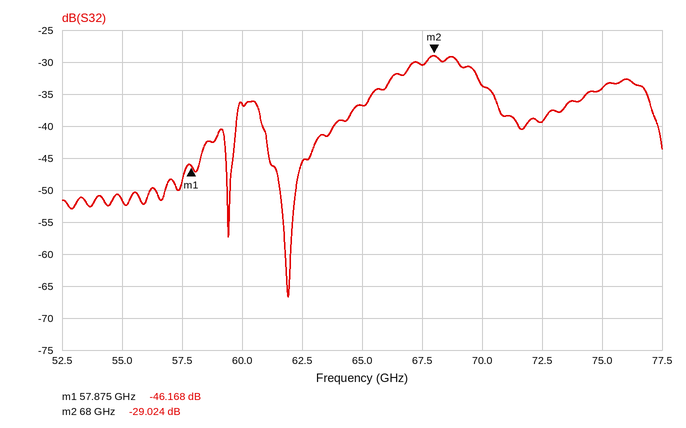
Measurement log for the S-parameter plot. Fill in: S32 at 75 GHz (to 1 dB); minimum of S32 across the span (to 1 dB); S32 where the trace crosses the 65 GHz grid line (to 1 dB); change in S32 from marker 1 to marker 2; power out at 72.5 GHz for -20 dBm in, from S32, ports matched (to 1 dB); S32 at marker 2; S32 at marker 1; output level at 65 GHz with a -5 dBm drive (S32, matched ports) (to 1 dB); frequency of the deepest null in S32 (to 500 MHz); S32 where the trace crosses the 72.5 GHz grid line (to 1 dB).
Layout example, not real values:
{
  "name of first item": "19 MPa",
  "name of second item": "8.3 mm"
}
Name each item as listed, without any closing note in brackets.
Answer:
{
  "S32 at 75 GHz": "-34 dB",
  "minimum of S32 across the span": "-67 dB",
  "S32 where the trace crosses the 65 GHz grid line": "-37 dB",
  "change in S32 from marker 1 to marker 2": "17.144 dB",
  "power out at 72.5 GHz for -20 dBm in, from S32, ports matched": "-59 dBm",
  "S32 at marker 2": "-29.024 dB",
  "S32 at marker 1": "-46.168 dB",
  "output level at 65 GHz with a -5 dBm drive (S32, matched ports)": "-42 dBm",
  "frequency of the deepest null in S32": "62.0 GHz",
  "S32 where the trace crosses the 72.5 GHz grid line": "-39 dB"
}
